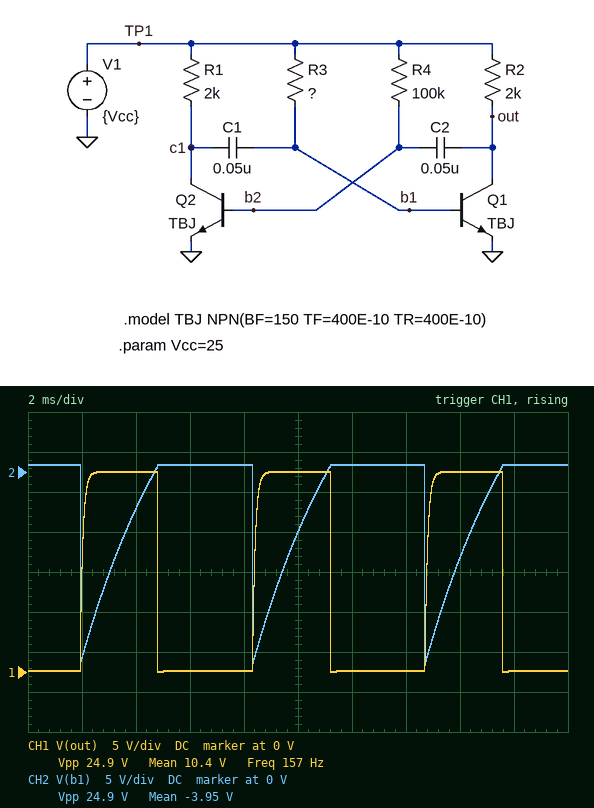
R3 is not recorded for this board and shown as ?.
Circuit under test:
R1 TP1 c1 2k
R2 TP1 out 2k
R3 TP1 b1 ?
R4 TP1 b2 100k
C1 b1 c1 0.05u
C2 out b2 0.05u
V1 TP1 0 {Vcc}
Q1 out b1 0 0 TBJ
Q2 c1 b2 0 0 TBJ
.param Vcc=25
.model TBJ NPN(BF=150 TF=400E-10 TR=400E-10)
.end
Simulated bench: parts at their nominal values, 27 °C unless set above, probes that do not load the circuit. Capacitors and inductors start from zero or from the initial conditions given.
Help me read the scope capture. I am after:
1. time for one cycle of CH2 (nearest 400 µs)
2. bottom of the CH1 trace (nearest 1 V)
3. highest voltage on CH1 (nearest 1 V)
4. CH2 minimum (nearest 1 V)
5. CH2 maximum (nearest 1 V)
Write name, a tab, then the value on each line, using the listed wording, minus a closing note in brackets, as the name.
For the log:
time for one cycle of CH2	6.4 ms
bottom of the CH1 trace	0 V
highest voltage on CH1	25 V
CH2 minimum	-24 V
CH2 maximum	1 V
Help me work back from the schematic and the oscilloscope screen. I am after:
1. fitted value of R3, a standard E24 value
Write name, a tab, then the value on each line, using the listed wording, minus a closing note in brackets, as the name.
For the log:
fitted value of R3, a standard E24 value	82 kΩ
